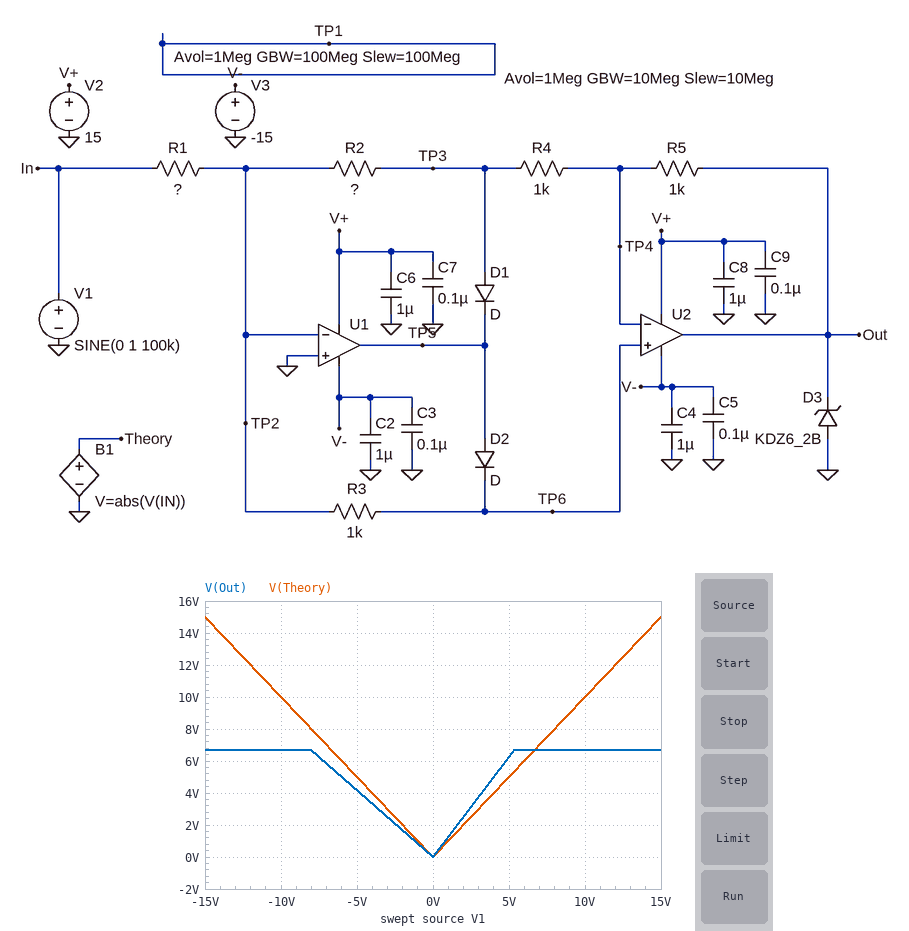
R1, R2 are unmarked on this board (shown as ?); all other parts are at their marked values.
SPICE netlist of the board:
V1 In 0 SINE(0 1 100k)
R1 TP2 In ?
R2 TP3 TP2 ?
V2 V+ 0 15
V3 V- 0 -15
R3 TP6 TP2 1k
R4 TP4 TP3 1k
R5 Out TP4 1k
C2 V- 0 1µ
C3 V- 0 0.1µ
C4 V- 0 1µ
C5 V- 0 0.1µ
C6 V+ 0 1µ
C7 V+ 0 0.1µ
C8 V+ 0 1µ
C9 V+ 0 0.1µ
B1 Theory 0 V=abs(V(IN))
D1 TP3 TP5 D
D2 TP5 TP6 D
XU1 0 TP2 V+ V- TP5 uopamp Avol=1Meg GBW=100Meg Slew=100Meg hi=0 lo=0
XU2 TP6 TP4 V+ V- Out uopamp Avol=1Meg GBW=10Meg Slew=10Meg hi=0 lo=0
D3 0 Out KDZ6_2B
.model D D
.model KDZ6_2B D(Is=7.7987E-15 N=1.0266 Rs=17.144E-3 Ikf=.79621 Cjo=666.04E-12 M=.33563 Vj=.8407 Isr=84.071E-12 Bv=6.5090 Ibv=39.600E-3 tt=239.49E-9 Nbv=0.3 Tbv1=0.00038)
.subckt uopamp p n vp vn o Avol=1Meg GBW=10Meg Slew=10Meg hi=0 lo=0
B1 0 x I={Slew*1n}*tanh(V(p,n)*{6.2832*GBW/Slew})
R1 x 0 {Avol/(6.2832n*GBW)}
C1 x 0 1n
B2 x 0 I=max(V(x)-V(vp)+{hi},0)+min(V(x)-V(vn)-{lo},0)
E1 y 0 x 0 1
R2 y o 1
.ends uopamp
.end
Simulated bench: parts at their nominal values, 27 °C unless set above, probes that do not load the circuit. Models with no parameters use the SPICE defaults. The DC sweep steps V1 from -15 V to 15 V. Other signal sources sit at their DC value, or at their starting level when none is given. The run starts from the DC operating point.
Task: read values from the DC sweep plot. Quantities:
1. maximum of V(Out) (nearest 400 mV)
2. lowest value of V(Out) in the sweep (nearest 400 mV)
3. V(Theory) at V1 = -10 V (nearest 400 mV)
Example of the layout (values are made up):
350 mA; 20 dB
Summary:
6.8 V; 0 V; 10.0 V
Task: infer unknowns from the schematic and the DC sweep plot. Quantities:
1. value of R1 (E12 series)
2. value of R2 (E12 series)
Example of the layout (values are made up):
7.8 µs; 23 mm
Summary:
1.2 kΩ; 1.5 kΩ
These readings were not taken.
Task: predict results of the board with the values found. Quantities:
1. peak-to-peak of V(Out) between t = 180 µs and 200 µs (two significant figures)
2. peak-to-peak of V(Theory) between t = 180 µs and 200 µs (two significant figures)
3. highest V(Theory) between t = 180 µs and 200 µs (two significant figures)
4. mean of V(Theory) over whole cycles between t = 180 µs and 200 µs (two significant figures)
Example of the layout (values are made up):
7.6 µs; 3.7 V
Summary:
1.3 V; 1.0 V; 1.0 V; 640 mV
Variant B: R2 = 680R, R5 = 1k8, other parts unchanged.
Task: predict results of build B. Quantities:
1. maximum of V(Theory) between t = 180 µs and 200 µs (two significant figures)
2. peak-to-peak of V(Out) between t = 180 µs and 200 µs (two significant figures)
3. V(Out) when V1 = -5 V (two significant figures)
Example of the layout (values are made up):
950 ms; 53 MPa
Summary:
1.0 V; 1.1 V; 5.4 V
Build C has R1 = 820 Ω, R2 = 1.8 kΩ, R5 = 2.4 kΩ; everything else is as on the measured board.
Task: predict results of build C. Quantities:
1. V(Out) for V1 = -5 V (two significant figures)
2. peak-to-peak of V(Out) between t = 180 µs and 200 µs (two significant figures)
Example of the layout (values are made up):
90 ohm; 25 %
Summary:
6.7 V; 5.3 V
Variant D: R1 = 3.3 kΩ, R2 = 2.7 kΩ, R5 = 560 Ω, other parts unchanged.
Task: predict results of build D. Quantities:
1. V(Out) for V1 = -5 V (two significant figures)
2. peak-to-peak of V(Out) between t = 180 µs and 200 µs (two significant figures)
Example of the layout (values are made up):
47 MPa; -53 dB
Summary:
1.4 V; 490 mV
